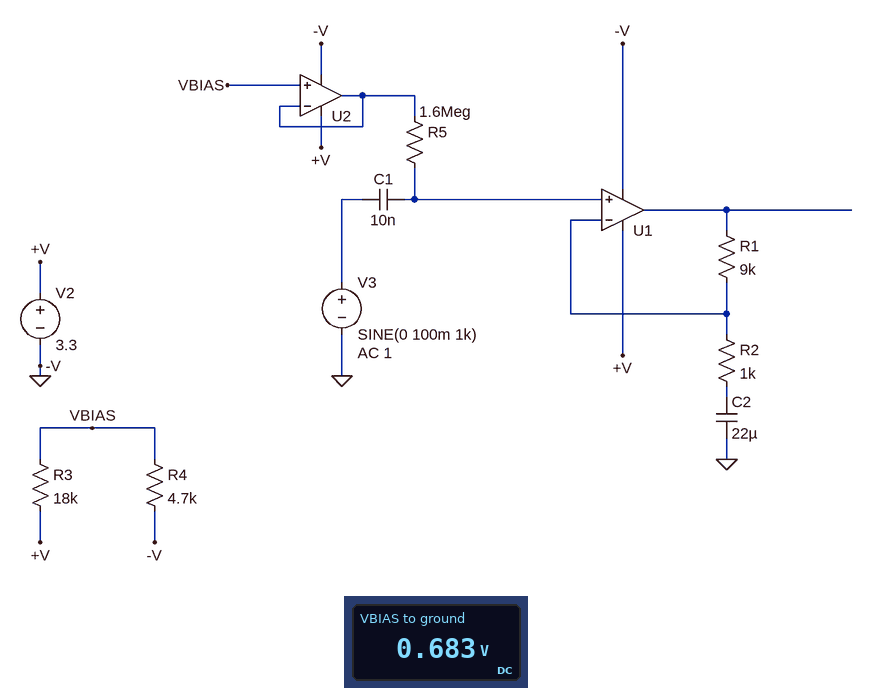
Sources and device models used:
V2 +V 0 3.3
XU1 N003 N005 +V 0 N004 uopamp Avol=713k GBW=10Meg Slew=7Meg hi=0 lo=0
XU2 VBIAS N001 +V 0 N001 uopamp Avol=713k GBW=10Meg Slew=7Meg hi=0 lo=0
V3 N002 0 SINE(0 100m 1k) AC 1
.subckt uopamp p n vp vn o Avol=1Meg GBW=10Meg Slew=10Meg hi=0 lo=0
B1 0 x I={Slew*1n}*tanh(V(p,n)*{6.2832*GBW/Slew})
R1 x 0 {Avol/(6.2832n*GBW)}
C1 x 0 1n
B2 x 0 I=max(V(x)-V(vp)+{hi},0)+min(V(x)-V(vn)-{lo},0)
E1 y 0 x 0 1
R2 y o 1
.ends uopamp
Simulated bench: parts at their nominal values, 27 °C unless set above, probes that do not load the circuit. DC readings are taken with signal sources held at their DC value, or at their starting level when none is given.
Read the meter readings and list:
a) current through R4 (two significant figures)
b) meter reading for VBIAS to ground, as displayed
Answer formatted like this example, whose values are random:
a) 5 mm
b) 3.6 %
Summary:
a) 150 µA
b) 0.683 V
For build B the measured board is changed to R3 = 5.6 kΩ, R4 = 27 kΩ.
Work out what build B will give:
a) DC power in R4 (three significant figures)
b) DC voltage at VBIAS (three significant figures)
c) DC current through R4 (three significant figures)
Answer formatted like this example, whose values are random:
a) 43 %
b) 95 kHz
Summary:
a) 277 µW
b) 2.73 V
c) 101 µA
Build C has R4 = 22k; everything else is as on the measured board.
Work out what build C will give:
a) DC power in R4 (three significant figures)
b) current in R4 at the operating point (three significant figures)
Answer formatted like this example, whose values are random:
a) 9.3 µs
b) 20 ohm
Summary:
a) 150 µW
b) 82.5 µA
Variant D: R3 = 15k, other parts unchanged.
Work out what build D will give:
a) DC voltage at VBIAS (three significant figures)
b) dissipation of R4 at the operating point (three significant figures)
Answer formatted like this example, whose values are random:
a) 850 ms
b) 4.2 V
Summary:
a) 787 mV
b) 132 µW
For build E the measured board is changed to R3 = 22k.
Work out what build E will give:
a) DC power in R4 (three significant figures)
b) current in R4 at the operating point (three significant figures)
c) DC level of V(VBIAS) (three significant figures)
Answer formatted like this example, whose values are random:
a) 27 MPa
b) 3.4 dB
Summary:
a) 71.8 µW
b) 124 µA
c) 581 mV
